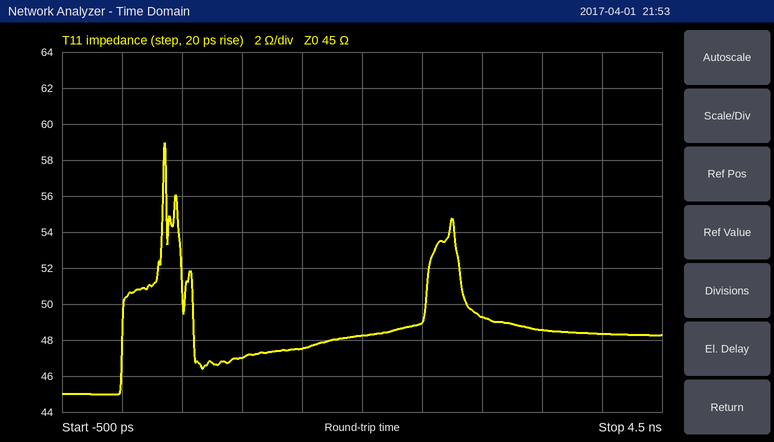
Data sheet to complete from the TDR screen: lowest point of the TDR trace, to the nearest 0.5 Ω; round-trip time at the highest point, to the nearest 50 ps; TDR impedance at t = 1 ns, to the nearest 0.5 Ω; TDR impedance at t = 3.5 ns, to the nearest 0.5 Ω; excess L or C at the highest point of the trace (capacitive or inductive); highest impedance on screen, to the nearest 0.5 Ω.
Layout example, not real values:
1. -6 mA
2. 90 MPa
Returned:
1. 45.0 Ω
2. 350 ps
3. 47.0 Ω
4. 48.5 Ω
5. inductive
6. 59.0 Ω
